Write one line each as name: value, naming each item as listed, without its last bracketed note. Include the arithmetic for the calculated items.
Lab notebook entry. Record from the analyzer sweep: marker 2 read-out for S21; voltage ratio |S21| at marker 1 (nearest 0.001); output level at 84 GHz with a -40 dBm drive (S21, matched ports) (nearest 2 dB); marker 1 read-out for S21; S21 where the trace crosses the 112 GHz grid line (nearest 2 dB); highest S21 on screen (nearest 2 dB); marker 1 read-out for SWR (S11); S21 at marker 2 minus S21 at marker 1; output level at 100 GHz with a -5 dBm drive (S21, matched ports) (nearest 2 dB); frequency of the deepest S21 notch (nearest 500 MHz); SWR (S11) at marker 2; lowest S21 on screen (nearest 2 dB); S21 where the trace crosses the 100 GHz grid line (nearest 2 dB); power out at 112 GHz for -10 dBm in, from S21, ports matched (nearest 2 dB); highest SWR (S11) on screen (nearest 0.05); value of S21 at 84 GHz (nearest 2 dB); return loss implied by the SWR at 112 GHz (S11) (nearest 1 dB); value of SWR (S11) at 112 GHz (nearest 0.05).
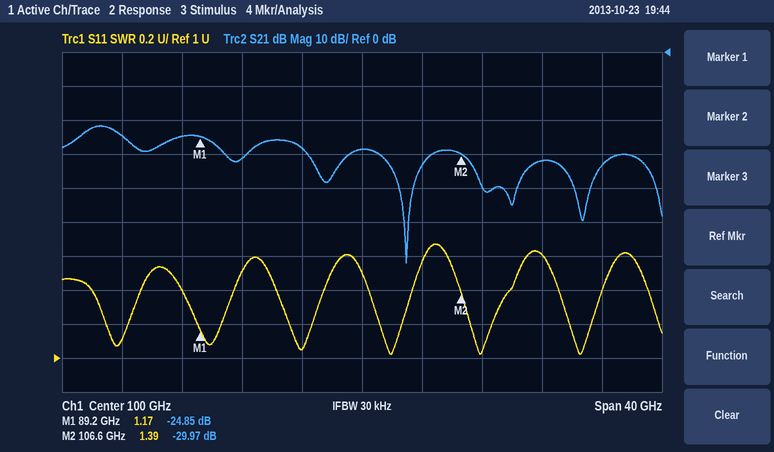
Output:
marker 2 read-out for S21: -29.97 dB
voltage ratio |S21| at marker 1: 10^(-24.85/20) ≈ 0.057
output level at 84 GHz with a -40 dBm drive (S21, matched ports): -40 dBm + (-24 dB) = -64 dBm
marker 1 read-out for S21: -24.85 dB
S21 where the trace crosses the 112 GHz grid line: -32 dB
highest S21 on screen: -22 dB
marker 1 read-out for SWR: 1.17
S21 at marker 2 minus S21 at marker 1: -29.97 − (-24.85) = -5.12 dB
output level at 100 GHz with a -5 dBm drive (S21, matched ports): -5 dBm + (-28 dB) = -34 dBm
frequency of the deepest S21 notch: 103.0 GHz
SWR (S11) at marker 2: 1.39
lowest S21 on screen: -62 dB
S21 where the trace crosses the 100 GHz grid line: -28 dB
power out at 112 GHz for -10 dBm in, from S21, ports matched: -10 dBm + (-32 dB) = -42 dBm
highest SWR (S11) on screen: 1.65
value of S21 at 84 GHz: -24 dB
return loss implied by the SWR at 112 GHz (S11): −20 log10((1.6 − 1)/(1.6 + 1)) ≈ 13 dB
value of SWR (S11) at 112 GHz: 1.60
